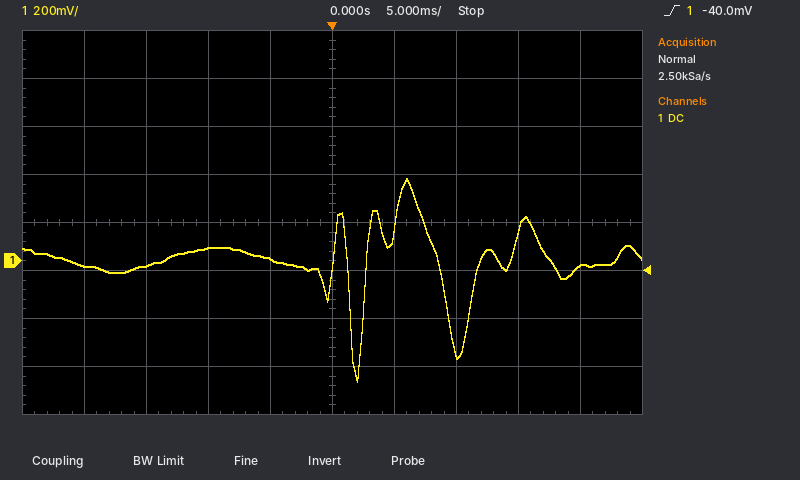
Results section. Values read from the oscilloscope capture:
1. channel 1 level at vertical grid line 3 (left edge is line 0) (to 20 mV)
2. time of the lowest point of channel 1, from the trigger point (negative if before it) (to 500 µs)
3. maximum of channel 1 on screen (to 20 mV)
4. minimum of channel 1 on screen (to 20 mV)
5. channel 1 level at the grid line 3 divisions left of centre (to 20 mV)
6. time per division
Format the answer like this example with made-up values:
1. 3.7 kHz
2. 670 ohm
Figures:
1. 60 mV
2. +2.0 ms
3. 340 mV
4. -500 mV
5. -20 mV
6. 5 ms
